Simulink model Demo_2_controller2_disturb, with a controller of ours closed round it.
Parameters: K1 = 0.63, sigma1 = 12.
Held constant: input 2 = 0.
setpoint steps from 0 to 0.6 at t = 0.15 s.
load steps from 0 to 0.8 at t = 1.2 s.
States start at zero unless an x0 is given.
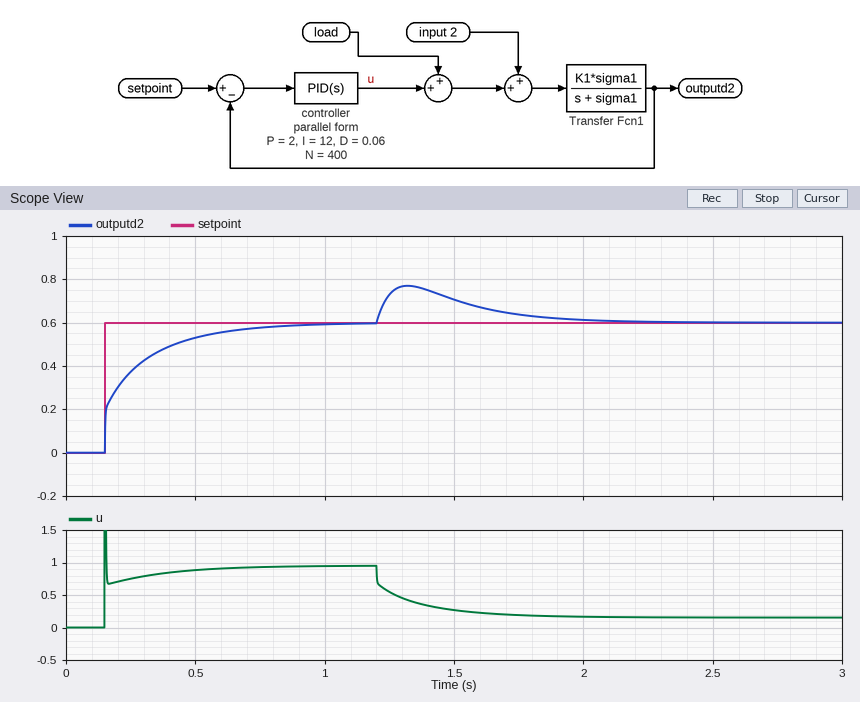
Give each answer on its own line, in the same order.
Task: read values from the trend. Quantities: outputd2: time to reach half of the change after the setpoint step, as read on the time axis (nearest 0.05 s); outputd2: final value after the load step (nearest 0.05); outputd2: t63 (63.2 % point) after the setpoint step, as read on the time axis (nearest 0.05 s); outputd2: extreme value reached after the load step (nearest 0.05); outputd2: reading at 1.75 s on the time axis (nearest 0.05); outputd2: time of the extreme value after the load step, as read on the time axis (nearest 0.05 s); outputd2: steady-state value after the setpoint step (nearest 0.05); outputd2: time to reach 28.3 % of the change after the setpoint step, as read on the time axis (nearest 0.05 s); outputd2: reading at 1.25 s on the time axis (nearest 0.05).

0.20 s
0.60
0.25 s
0.75
0.65
1.30 s
0.60
0.15 s
0.75
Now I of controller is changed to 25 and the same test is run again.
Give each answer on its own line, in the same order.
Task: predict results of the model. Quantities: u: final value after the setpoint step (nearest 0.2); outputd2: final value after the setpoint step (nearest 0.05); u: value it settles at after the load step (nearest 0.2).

1.0
0.60
0.2
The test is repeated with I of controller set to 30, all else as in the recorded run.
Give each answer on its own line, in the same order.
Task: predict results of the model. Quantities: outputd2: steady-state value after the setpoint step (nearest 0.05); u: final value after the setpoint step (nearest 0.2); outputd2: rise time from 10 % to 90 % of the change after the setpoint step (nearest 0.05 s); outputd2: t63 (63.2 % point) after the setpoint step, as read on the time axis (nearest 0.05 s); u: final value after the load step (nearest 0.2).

0.60
1.0
0.15 s
0.20 s
0.2
